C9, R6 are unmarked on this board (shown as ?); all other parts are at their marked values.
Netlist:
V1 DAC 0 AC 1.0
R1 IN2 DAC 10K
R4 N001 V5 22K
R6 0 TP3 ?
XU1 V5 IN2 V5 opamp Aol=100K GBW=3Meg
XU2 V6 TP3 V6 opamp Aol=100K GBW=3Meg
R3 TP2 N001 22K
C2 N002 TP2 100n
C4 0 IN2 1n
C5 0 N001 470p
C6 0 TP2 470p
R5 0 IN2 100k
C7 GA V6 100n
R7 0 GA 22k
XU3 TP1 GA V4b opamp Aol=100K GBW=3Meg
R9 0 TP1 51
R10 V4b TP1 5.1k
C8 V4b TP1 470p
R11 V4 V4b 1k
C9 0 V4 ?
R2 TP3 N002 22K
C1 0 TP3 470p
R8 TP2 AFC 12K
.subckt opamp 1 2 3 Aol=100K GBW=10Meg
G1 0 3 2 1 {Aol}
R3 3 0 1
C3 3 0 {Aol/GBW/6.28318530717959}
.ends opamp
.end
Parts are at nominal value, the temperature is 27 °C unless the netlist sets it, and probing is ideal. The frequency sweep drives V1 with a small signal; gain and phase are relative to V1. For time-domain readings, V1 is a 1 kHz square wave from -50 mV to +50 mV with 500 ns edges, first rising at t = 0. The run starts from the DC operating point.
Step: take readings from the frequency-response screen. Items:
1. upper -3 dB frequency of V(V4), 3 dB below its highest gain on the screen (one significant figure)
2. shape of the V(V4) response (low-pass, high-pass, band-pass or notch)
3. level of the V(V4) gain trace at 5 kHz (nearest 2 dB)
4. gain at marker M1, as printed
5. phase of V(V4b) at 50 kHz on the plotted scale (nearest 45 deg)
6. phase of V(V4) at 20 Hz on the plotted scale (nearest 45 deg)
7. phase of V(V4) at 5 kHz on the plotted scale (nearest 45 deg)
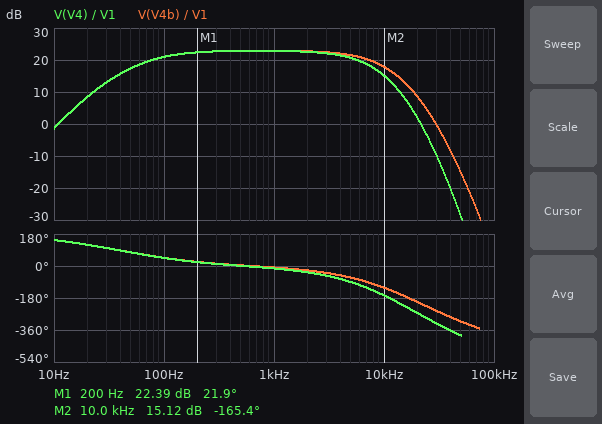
6 kHz
band-pass
20 dB
22.39 dB
-315 deg
135 deg
-90 deg
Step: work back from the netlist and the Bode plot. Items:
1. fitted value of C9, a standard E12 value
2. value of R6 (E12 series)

15 nF
12 kΩ
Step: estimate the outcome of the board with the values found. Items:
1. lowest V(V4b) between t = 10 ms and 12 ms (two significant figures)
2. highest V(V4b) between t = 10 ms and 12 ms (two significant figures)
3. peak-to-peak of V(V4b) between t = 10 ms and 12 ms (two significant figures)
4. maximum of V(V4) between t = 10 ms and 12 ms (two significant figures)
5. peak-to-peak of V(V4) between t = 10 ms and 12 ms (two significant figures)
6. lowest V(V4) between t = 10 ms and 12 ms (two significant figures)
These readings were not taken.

-830 mV
710 mV
1.5 V
700 mV
1.5 V
-820 mV
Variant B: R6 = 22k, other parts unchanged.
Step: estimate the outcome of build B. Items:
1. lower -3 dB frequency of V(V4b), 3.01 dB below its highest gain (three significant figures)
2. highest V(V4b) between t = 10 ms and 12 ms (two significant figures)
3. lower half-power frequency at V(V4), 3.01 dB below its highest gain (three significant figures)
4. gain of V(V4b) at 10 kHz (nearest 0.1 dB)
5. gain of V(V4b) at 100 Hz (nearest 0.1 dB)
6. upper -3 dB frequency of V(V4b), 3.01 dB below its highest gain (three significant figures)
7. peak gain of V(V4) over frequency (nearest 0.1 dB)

75.0 Hz
1.1 V
74.7 Hz
21.0 dB
25.2 dB
6.57 kHz
27.1 dB
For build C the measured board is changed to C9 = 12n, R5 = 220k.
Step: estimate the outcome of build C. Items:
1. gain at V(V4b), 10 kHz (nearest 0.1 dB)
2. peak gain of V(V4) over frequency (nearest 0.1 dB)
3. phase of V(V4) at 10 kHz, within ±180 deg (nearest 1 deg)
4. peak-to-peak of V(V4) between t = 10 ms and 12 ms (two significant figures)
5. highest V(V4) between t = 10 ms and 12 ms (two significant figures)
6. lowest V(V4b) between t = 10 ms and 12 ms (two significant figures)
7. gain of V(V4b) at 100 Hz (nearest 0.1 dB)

18.2 dB
23.3 dB
-160 deg
1.6 V
740 mV
-870 mV
21.4 dB
